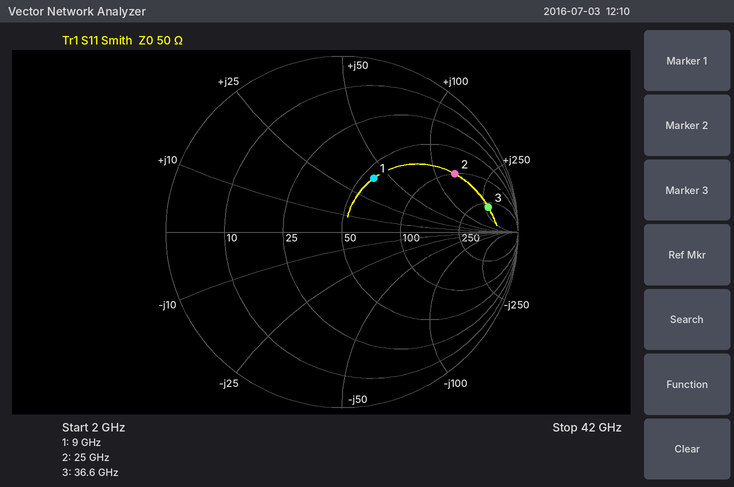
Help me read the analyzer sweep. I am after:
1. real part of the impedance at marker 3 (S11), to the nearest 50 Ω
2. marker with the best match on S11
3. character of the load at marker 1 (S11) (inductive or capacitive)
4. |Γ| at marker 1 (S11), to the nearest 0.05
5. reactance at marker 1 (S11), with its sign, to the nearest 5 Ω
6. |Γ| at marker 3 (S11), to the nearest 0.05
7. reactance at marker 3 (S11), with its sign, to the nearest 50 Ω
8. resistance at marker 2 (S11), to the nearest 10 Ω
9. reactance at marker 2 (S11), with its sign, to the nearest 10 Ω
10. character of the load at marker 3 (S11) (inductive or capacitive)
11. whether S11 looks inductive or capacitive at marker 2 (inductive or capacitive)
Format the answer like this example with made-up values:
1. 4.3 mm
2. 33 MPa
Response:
1. 300 Ω
2. marker 1
3. inductive
4. 0.35
5. +40 Ω
6. 0.85
7. +300 Ω
8. 100 Ω
9. +140 Ω
10. inductive
11. inductive
